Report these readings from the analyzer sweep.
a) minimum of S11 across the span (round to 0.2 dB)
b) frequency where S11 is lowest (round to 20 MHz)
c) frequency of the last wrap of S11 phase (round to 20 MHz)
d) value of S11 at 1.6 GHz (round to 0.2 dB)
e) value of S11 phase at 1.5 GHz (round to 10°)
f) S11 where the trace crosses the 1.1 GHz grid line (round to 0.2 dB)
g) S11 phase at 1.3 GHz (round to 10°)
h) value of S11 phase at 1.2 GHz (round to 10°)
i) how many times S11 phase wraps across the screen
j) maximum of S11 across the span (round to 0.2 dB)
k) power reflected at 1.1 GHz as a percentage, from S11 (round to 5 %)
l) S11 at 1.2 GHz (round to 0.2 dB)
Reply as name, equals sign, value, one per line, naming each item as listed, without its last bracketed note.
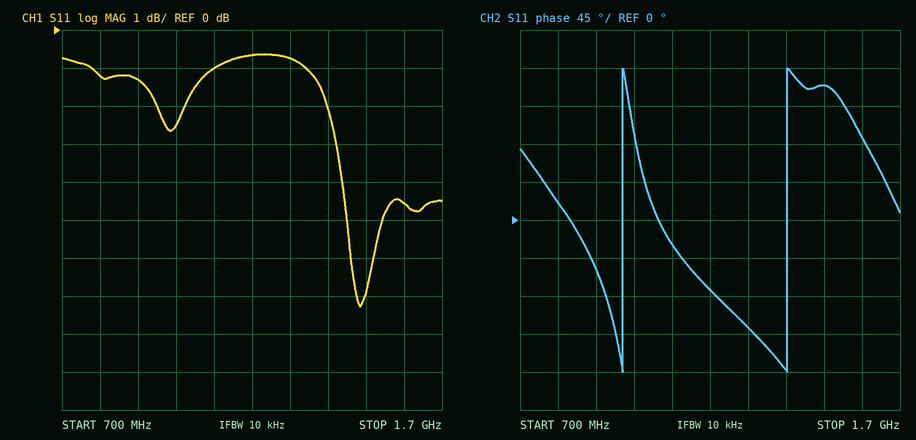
minimum of S11 across the span = -7.2 dB
frequency where S11 is lowest = 1.48 GHz
frequency of the last wrap of S11 phase = 1.40 GHz
value of S11 at 1.6 GHz = -4.6 dB
value of S11 phase at 1.5 GHz = 160°
S11 where the trace crosses the 1.1 GHz grid line = -1.0 dB
S11 phase at 1.3 GHz = -130°
value of S11 phase at 1.2 GHz = -80°
how many times S11 phase wraps across the screen = 2
maximum of S11 across the span = -0.6 dB
power reflected at 1.1 GHz as a percentage, from S11 = 80 %
S11 at 1.2 GHz = -0.6 dB
